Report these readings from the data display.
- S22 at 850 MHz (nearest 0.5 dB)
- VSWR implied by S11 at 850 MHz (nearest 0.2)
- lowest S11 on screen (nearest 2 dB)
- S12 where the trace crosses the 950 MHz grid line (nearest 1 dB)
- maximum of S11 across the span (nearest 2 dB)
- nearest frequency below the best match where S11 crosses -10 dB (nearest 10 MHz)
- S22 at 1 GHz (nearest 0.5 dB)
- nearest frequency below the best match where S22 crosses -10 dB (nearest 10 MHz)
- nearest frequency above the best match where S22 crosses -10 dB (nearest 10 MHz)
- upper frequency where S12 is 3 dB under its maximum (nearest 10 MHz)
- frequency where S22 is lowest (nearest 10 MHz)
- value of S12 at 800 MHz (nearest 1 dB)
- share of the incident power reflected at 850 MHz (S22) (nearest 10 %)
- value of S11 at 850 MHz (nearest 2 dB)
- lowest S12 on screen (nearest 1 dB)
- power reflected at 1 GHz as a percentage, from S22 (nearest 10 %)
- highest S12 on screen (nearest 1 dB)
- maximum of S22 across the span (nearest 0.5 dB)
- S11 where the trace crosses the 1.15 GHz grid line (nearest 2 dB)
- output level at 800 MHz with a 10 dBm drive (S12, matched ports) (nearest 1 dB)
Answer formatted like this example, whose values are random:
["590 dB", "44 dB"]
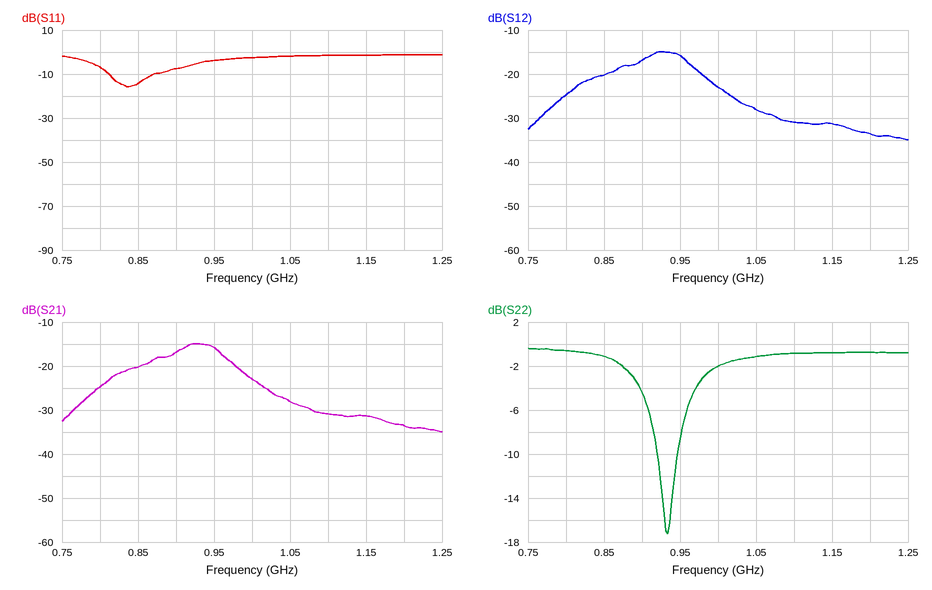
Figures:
["-1.0 dB", "1.4", "-16 dB", "-16 dB", "-2 dB", "810 MHz", "-2.0 dB", "920 MHz", "950 MHz", "960 MHz", "930 MHz", "-25 dB", "80 %", "-14 dB", "-35 dB", "60 %", "-15 dB", "-0.5 dB", "-2 dB", "-15 dBm"]
